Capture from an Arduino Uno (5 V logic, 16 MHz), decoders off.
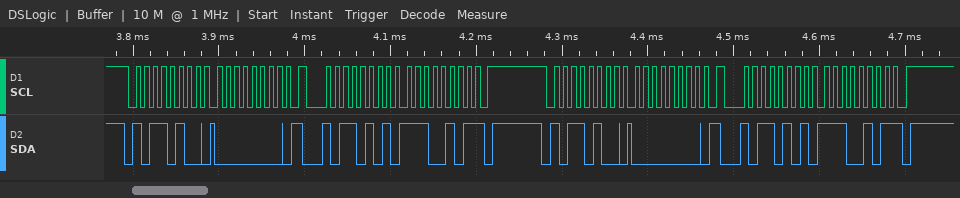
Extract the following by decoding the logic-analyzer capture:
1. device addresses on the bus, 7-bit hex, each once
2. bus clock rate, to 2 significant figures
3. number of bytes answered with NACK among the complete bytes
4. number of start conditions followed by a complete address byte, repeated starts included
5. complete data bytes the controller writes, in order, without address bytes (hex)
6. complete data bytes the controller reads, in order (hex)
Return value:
0x5A
100 kHz
2
4
00 00
E5 E5
